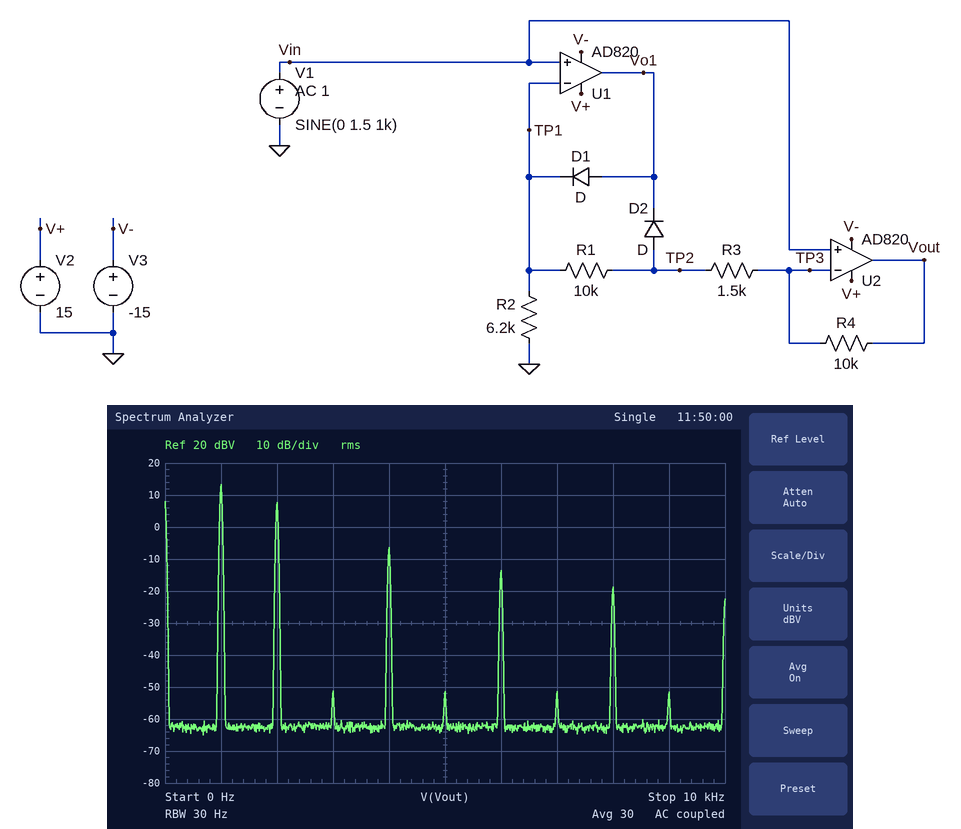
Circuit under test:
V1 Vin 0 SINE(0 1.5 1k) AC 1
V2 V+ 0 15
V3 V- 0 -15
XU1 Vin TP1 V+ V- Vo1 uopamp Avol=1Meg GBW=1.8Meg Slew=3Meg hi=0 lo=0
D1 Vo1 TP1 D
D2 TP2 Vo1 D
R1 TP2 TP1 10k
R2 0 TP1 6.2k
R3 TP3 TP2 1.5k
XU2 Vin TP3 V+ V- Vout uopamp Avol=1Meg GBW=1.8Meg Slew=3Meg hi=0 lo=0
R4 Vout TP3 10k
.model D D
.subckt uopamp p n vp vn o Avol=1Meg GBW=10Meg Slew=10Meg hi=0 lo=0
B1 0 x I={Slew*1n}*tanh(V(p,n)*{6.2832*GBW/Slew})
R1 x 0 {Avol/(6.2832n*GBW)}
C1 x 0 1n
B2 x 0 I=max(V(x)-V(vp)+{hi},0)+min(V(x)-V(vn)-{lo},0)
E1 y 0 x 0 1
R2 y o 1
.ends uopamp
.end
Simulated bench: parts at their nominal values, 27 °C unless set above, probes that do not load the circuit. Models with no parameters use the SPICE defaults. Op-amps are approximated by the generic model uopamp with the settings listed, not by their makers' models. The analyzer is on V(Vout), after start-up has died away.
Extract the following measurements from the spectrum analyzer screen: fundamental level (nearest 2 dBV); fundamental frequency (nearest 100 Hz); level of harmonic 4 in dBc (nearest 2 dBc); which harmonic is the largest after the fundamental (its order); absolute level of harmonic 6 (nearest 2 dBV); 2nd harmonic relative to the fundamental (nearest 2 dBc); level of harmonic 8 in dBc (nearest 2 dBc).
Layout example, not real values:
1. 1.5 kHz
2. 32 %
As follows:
1. 14 dBV
2. 1.0 kHz
3. -20 dBc
4. 2
5. -14 dBV
6. -6 dBc
7. -32 dBc
